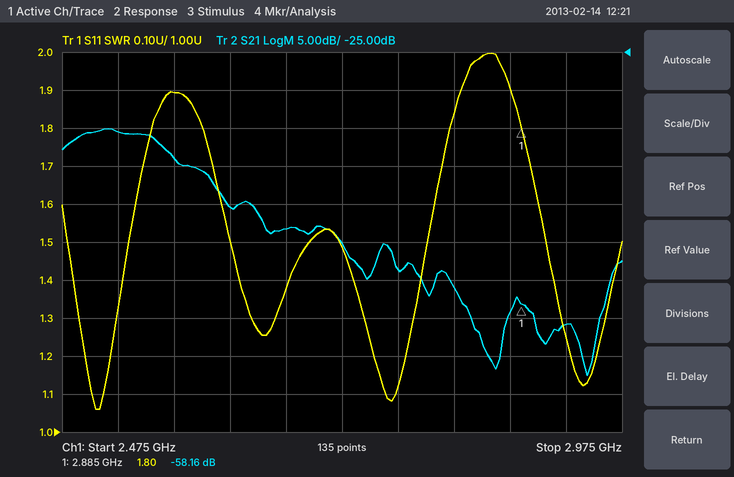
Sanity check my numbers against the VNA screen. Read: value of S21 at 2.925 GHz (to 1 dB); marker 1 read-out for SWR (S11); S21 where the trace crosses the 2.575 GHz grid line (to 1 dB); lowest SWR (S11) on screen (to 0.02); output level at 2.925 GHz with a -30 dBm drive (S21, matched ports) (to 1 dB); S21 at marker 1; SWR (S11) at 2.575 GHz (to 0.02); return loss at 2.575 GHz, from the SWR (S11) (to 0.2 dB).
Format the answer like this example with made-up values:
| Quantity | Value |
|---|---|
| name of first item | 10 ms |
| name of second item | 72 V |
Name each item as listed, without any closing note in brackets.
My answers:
| Quantity | Value |
|---|---|
| value of S21 at 2.925 GHz | -61 dB |
| marker 1 read-out for SWR | 1.80 |
| S21 where the trace crosses the 2.575 GHz grid line | -39 dB |
| lowest SWR (S11) on screen | 1.06 |
| output level at 2.925 GHz with a -30 dBm drive (S21, matched ports) | -91 dBm |
| S21 at marker 1 | -58.16 dB |
| SWR (S11) at 2.575 GHz | 1.90 |
| return loss at 2.575 GHz, from the SWR (S11) | 10.2 dB |
